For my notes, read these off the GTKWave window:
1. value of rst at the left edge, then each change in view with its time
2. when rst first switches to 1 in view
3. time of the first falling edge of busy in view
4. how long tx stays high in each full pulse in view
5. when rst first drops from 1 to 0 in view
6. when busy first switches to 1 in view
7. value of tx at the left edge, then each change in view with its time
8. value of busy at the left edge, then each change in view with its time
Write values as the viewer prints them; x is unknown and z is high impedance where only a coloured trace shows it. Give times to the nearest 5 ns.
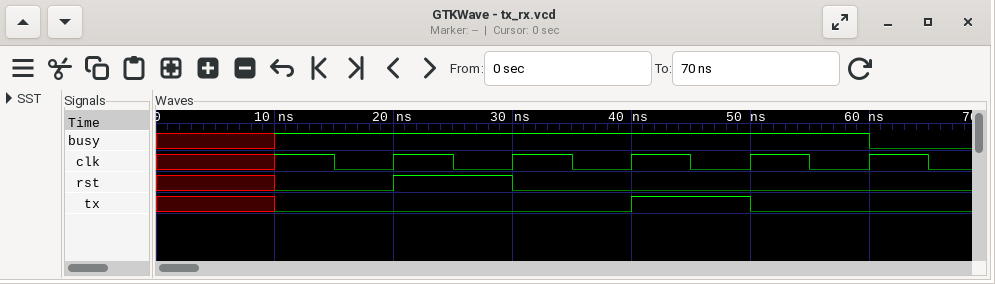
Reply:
x, 0 at 10 ns, 1 at 20 ns, 0 at 30 ns
20 ns
60 ns
10 ns
30 ns
10 ns
x, 0 at 10 ns, 1 at 40 ns, 0 at 50 ns
x, 1 at 10 ns, 0 at 60 ns
